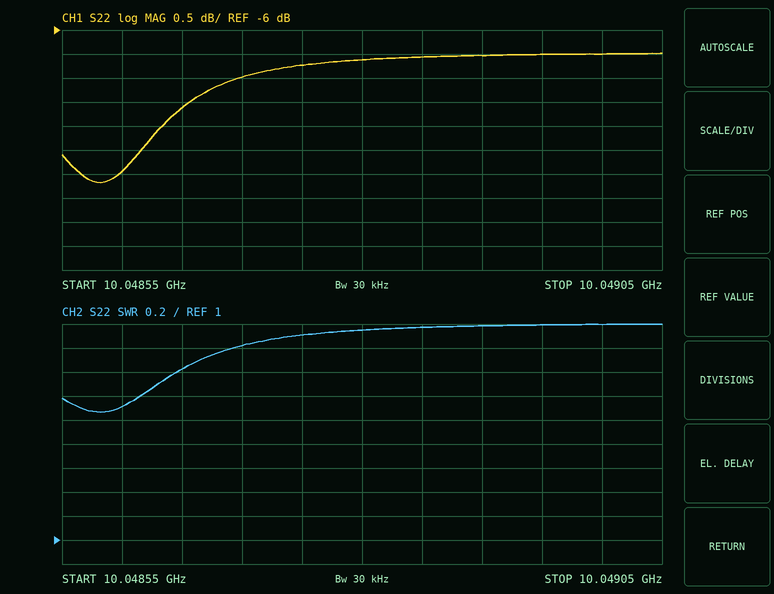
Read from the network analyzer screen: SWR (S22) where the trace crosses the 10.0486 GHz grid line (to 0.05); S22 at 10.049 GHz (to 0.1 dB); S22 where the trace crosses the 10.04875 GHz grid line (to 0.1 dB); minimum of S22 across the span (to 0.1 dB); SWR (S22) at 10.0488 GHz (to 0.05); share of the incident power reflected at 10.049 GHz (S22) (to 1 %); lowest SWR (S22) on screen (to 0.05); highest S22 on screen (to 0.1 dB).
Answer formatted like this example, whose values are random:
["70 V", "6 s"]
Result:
["2.10", "-6.5 dB", "-6.7 dB", "-9.2 dB", "2.75", "22 %", "2.05", "-6.5 dB"]
